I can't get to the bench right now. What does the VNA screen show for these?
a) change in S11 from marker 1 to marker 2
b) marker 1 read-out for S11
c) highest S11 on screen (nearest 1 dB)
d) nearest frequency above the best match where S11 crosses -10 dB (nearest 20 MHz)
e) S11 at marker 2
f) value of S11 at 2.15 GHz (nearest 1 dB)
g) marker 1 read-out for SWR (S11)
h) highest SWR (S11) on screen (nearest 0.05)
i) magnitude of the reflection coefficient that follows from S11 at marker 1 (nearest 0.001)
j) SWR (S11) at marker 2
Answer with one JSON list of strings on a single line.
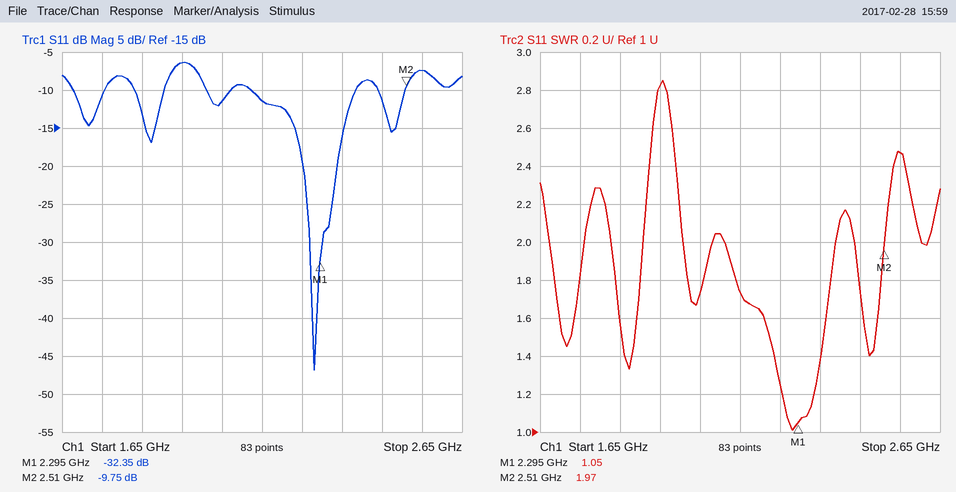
["22.60 dB", "-32.35 dB", "-6 dB", "2.38 GHz", "-9.75 dB", "-11 dB", "1.05", "2.85", "0.024", "1.97"]
